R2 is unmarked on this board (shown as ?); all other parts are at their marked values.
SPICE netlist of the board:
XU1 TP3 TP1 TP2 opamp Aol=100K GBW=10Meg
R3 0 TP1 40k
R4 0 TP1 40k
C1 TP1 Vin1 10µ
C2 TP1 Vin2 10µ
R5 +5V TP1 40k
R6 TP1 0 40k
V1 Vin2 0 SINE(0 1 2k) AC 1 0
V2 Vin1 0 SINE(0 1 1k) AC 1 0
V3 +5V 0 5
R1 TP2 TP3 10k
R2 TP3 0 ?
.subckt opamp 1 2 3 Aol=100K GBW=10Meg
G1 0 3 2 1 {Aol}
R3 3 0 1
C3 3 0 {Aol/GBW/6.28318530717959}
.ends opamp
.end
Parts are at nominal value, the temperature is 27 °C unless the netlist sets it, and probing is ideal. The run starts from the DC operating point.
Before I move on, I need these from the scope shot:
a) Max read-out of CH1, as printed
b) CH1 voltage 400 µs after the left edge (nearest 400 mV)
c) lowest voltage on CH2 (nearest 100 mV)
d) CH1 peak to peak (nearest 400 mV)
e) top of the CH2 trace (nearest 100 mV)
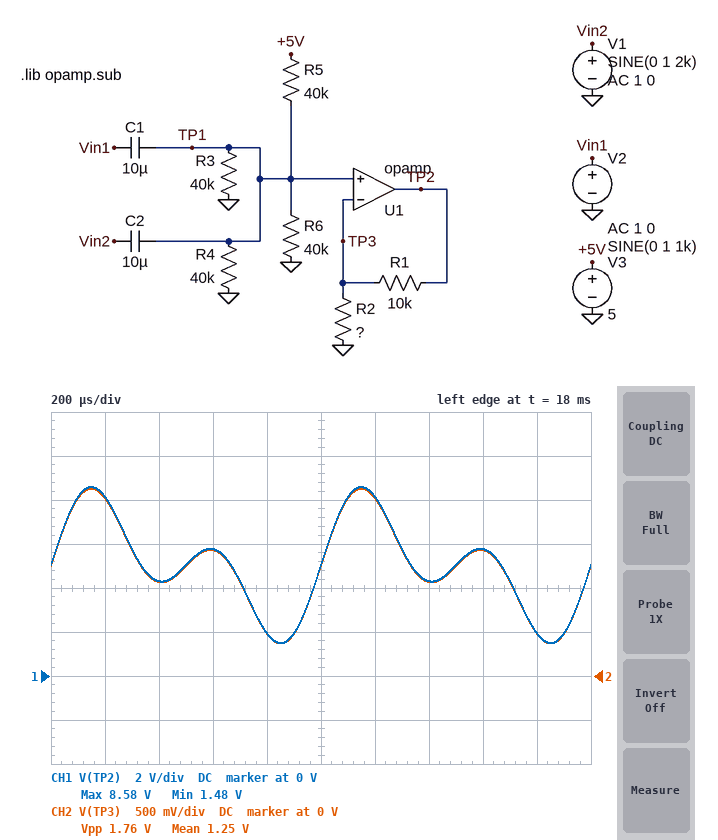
8.58 V
4.4 V
400 mV
7.2 V
2.1 V
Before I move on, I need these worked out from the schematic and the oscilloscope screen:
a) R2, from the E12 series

3.3 kΩ
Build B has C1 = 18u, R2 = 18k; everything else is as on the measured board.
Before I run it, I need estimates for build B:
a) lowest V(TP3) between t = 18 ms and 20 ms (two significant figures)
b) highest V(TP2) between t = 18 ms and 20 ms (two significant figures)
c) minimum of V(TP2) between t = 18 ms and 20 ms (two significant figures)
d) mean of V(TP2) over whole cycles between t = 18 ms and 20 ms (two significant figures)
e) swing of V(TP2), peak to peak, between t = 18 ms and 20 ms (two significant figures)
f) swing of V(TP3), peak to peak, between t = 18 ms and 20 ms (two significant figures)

380 mV
3.3 V
600 mV
1.9 V
2.7 V
1.7 V
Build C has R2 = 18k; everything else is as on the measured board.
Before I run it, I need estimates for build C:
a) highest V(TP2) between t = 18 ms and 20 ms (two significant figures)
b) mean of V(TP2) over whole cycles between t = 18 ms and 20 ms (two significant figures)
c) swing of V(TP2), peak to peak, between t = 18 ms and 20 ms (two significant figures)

3.3 V
1.9 V
2.7 V
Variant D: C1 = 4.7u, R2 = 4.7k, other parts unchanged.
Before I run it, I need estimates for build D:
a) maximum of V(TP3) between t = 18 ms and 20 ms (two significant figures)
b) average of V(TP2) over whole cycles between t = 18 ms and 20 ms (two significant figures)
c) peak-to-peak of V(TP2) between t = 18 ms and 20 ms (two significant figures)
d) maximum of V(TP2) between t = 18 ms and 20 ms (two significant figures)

2.2 V
3.9 V
5.7 V
6.8 V
